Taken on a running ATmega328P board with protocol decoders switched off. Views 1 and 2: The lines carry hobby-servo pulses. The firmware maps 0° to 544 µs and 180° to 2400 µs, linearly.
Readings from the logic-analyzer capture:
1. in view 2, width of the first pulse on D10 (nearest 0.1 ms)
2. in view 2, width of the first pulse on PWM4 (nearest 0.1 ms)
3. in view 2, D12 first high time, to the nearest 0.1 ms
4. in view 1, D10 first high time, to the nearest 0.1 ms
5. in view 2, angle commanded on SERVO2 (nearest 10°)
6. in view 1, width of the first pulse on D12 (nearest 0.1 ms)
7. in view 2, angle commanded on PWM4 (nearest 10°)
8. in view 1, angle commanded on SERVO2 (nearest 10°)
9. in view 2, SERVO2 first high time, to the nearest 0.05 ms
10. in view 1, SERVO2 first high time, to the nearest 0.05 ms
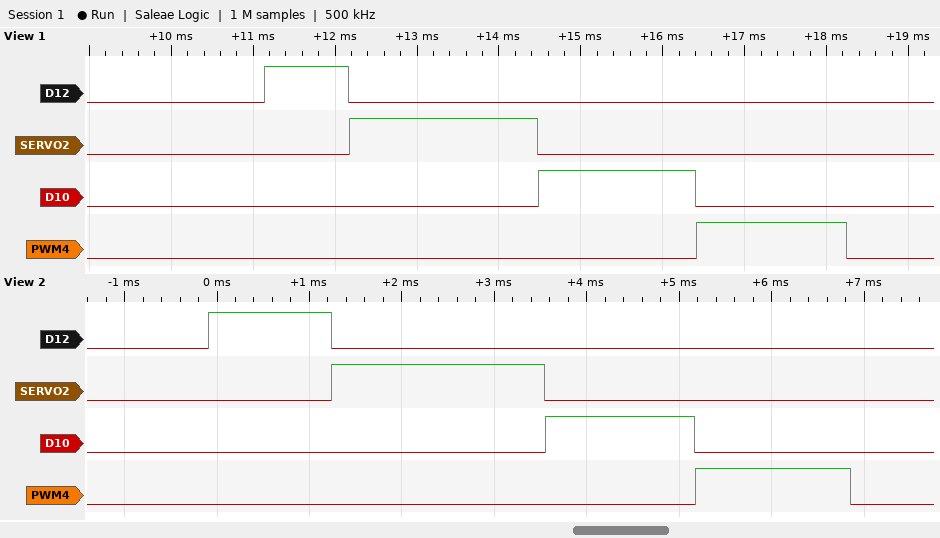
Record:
1.6 ms
1.7 ms
1.3 ms
1.9 ms
170°
1.0 ms
110°
170°
2.30 ms
2.30 ms
